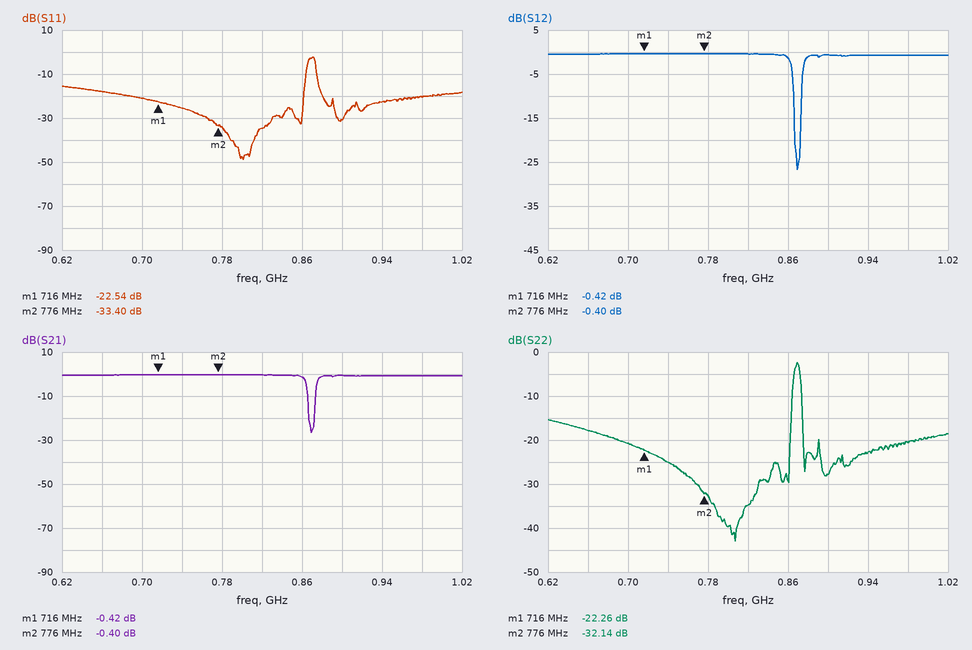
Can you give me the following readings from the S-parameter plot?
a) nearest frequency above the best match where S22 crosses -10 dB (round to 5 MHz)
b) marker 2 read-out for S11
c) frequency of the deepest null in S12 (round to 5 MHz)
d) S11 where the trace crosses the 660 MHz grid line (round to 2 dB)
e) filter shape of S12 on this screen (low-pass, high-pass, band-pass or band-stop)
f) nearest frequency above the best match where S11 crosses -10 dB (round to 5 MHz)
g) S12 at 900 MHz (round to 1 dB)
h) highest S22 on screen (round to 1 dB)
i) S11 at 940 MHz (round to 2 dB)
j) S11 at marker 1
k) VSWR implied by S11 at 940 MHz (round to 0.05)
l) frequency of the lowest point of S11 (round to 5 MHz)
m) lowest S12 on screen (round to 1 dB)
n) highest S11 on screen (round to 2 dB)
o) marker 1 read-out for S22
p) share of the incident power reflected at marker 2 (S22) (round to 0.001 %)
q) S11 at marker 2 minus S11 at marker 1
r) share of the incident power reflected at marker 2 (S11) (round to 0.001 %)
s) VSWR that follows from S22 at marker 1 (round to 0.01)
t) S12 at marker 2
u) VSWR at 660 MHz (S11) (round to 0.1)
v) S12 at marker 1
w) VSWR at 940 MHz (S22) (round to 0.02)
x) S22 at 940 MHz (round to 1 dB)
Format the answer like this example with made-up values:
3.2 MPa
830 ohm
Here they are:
865 MHz
-33.40 dB
870 MHz
-18 dB
band-stop
865 MHz
-1 dB
-2 dB
-22 dB
-22.54 dB
1.15
800 MHz
-27 dB
-2 dB
-22.26 dB
0.061 %
-10.86 dB
0.046 %
1.17
-0.40 dB
1.3
-0.42 dB
1.16
-23 dB
